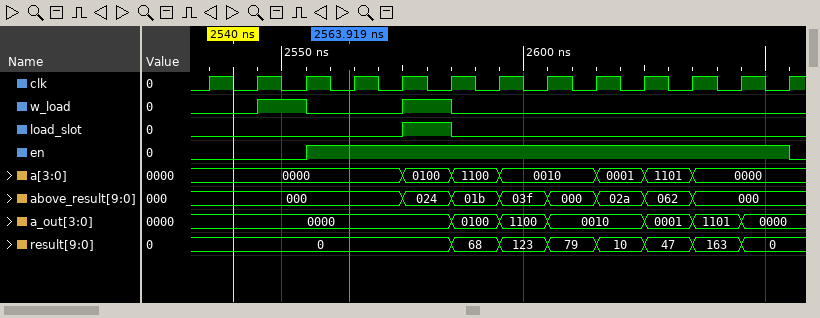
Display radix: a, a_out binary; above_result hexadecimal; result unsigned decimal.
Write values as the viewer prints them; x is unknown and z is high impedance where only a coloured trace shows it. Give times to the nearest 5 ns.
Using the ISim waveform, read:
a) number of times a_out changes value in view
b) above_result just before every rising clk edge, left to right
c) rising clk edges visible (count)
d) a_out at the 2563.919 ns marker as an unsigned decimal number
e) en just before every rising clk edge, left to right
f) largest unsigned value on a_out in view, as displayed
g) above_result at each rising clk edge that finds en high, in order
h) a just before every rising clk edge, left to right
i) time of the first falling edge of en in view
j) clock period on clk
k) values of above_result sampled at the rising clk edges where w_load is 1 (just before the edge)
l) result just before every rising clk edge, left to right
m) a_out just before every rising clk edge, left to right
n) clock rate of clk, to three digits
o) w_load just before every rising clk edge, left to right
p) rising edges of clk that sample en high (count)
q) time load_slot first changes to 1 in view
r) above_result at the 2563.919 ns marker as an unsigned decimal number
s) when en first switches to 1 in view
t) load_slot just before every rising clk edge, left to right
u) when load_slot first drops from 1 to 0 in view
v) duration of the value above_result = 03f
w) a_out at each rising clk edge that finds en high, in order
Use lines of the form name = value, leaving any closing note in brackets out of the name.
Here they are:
number of times a_out changes value in view = 6
above_result just before every rising clk edge, left to right = 000, 000, 000, 000, 000, 024, 01b, 03f, 000, 02a, 062, 000, 000
rising clk edges visible = 13
a_out at the 2563.919 ns marker as an unsigned decimal number = 0
en just before every rising clk edge, left to right = 0 0 0 1 1 1 1 1 1 1 1 1 1
largest unsigned value on a_out in view, as displayed = 1101
above_result at each rising clk edge that finds en high, in order = 000, 000, 024, 01b, 03f, 000, 02a, 062, 000, 000
a just before every rising clk edge, left to right = 0000, 0000, 0000, 0000, 0000, 0100, 1100, 0010, 0010, 0001, 1101, 0000, 0000
time of the first falling edge of en in view = 2655 ns
clock period on clk = 10 ns
values of above_result sampled at the rising clk edges where w_load is 1 = 000, 024
result just before every rising clk edge, left to right = 0, 0, 0, 0, 0, 0, 68, 123, 79, 10, 47, 163, 0
a_out just before every rising clk edge, left to right = 0000, 0000, 0000, 0000, 0000, 0000, 0100, 1100, 0010, 0010, 0001, 1101, 0000
clock rate of clk, to three digits = 100 MHz
w_load just before every rising clk edge, left to right = 0 0 1 0 0 1 0 0 0 0 0 0 0
rising edges of clk that sample en high = 10
time load_slot first changes to 1 in view = 2575 ns
above_result at the 2563.919 ns marker as an unsigned decimal number = 0
when en first switches to 1 in view = 2555 ns
load_slot just before every rising clk edge, left to right = 0 0 0 0 0 1 0 0 0 0 0 0 0
when load_slot first drops from 1 to 0 in view = 2585 ns
duration of the value above_result = 03f = 10 ns
a_out at each rising clk edge that finds en high, in order = 0000, 0000, 0000, 0100, 1100, 0010, 0010, 0001, 1101, 0000
